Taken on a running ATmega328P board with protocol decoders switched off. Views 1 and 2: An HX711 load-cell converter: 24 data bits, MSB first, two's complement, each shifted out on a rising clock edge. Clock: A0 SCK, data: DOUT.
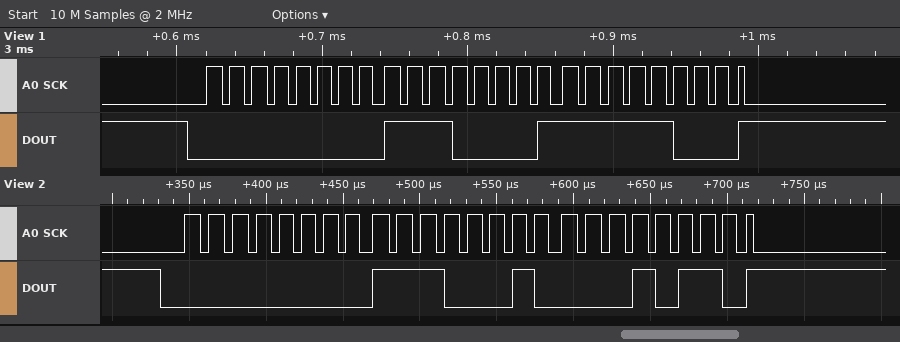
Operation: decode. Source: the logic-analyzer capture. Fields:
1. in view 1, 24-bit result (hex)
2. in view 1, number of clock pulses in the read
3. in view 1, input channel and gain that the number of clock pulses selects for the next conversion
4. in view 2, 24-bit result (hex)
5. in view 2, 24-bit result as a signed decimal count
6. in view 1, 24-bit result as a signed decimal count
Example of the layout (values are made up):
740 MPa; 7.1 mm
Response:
0x00E1F8; 25; channel A, gain 128; 0x00E216; 57878; 57848
